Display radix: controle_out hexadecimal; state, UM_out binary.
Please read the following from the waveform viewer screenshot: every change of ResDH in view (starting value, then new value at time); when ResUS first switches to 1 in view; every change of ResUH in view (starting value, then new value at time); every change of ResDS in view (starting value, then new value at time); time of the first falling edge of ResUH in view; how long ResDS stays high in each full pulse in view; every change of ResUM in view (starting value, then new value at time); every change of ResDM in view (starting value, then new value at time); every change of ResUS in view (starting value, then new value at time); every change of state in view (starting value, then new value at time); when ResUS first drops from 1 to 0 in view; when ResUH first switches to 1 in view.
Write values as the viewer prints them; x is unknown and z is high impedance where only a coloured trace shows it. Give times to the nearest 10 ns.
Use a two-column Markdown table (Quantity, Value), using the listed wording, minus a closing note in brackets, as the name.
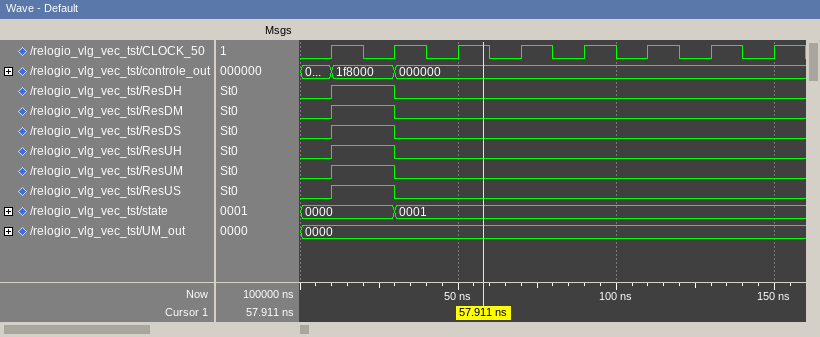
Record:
| Quantity | Value |
|---|---|
| every change of ResDH in view | 0, 1 at 10 ns, 0 at 30 ns |
| when ResUS first switches to 1 in view | 10 ns |
| every change of ResUH in view | 0, 1 at 10 ns, 0 at 30 ns |
| every change of ResDS in view | 0, 1 at 10 ns, 0 at 30 ns |
| time of the first falling edge of ResUH in view | 30 ns |
| how long ResDS stays high in each full pulse in view | 20 ns |
| every change of ResUM in view | 0, 1 at 10 ns, 0 at 30 ns |
| every change of ResDM in view | 0, 1 at 10 ns, 0 at 30 ns |
| every change of ResUS in view | 0, 1 at 10 ns, 0 at 30 ns |
| every change of state in view | 0000, 0001 at 30 ns |
| when ResUS first drops from 1 to 0 in view | 30 ns |
| when ResUH first switches to 1 in view | 10 ns |
